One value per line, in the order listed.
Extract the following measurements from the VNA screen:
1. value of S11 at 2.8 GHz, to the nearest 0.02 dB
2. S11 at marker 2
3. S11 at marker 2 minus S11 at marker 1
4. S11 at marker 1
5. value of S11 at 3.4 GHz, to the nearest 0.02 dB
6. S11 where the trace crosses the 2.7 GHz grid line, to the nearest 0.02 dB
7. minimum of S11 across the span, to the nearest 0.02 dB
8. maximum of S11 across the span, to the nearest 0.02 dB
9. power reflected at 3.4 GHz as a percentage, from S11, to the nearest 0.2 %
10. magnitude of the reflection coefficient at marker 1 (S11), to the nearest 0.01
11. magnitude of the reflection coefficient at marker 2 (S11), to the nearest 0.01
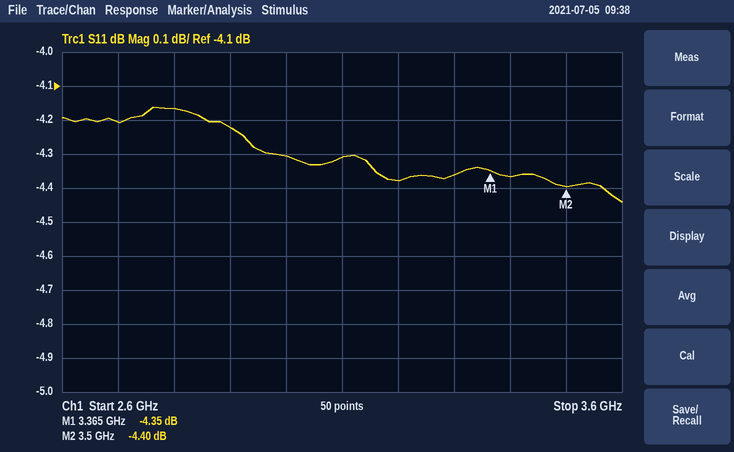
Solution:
-4.16 dB
-4.40 dB
-0.05 dB
-4.35 dB
-4.36 dB
-4.20 dB
-4.44 dB
-4.16 dB
36.6 %
0.61
0.60
